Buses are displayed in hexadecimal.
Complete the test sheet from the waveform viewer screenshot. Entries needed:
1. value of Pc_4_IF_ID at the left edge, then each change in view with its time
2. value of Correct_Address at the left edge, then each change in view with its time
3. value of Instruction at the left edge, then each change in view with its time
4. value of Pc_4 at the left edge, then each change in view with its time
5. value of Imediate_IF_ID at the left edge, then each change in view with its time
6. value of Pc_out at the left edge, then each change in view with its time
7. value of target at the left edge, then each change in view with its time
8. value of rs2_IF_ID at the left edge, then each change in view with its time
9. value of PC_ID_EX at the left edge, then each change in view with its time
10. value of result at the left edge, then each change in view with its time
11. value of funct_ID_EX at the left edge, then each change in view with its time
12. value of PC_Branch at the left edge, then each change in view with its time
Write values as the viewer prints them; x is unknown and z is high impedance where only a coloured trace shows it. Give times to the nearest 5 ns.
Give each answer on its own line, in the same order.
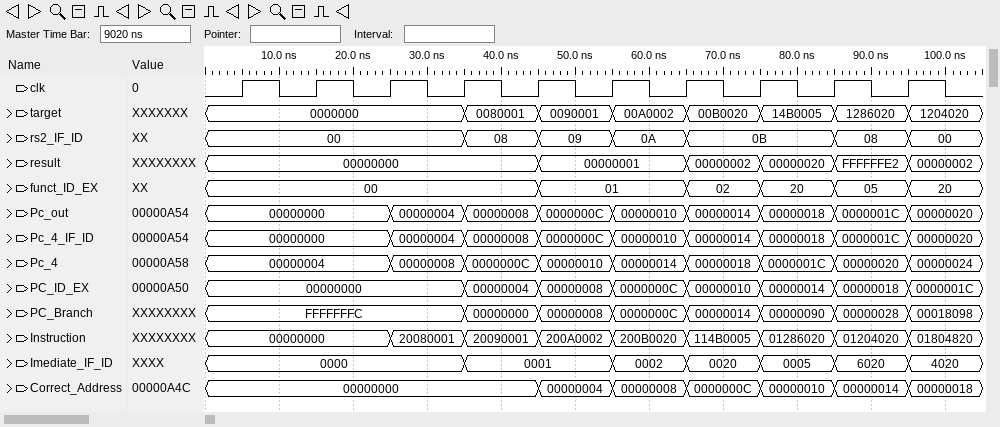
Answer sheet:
00000000, 00000004 at 25 ns, 00000008 at 35 ns, 0000000C at 45 ns, 00000010 at 55 ns, 00000014 at 65 ns, 00000018 at 75 ns, 0000001C at 85 ns, 00000020 at 95 ns
00000000, 00000004 at 45 ns, 00000008 at 55 ns, 0000000C at 65 ns, 00000010 at 75 ns, 00000014 at 85 ns, 00000018 at 95 ns
00000000, 20080001 at 25 ns, 20090001 at 35 ns, 200A0002 at 45 ns, 200B0020 at 55 ns, 114B0005 at 65 ns, 01286020 at 75 ns, 01204020 at 85 ns, 01804820 at 95 ns
00000004, 00000008 at 25 ns, 0000000C at 35 ns, 00000010 at 45 ns, 00000014 at 55 ns, 00000018 at 65 ns, 0000001C at 75 ns, 00000020 at 85 ns, 00000024 at 95 ns
0000, 0001 at 35 ns, 0002 at 55 ns, 0020 at 65 ns, 0005 at 75 ns, 6020 at 85 ns, 4020 at 95 ns
00000000, 00000004 at 25 ns, 00000008 at 35 ns, 0000000C at 45 ns, 00000010 at 55 ns, 00000014 at 65 ns, 00000018 at 75 ns, 0000001C at 85 ns, 00000020 at 95 ns
0000000, 0080001 at 35 ns, 0090001 at 45 ns, 00A0002 at 55 ns, 00B0020 at 65 ns, 14B0005 at 75 ns, 1286020 at 85 ns, 1204020 at 95 ns
00, 08 at 35 ns, 09 at 45 ns, 0A at 55 ns, 0B at 65 ns, 08 at 85 ns, 00 at 95 ns
00000000, 00000004 at 35 ns, 00000008 at 45 ns, 0000000C at 55 ns, 00000010 at 65 ns, 00000014 at 75 ns, 00000018 at 85 ns, 0000001C at 95 ns
00000000, 00000001 at 45 ns, 00000002 at 65 ns, 00000020 at 75 ns, FFFFFFE2 at 85 ns, 00000002 at 95 ns
00, 01 at 45 ns, 02 at 65 ns, 20 at 75 ns, 05 at 85 ns, 20 at 95 ns
FFFFFFFC, 00000000 at 35 ns, 00000008 at 45 ns, 0000000C at 55 ns, 00000014 at 65 ns, 00000090 at 75 ns, 00000028 at 85 ns, 00018098 at 95 ns
